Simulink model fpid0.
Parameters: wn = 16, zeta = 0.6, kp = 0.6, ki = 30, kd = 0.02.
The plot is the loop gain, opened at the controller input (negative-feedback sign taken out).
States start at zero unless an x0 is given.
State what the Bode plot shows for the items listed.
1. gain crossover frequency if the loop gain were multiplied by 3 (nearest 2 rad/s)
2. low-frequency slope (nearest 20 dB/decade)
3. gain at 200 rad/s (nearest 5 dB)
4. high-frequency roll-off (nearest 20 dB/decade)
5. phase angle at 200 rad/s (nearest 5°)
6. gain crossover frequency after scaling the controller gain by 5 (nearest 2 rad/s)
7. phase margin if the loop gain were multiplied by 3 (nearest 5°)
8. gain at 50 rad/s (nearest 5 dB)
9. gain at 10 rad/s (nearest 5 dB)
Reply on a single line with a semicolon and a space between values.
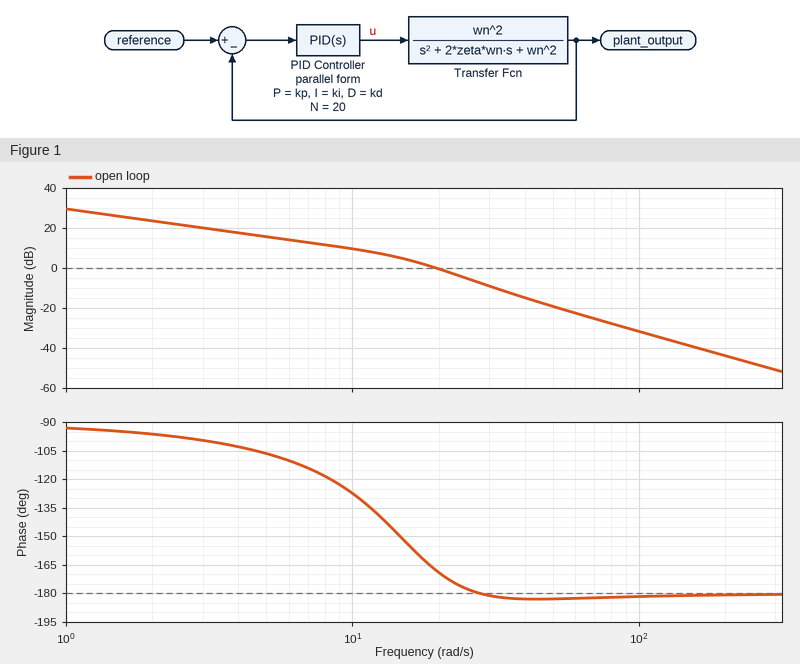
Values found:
30 rad/s; -20 dB/decade; -45 dB; -40 dB/decade; -180°; 38 rad/s; 0°; -20 dB; 10 dB
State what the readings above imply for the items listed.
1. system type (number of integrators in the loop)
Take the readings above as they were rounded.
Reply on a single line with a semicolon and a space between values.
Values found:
1
